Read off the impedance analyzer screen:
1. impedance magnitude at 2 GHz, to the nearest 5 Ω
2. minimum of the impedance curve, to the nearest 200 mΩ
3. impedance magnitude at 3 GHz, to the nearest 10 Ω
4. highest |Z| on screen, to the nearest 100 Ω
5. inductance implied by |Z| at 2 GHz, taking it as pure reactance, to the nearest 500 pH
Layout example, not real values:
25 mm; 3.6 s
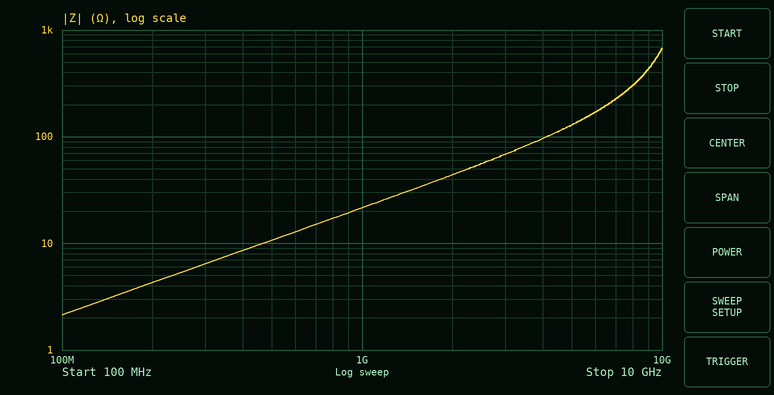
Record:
45 Ω; 2.2 Ω; 70 Ω; 700 Ω; 3.5 nH
